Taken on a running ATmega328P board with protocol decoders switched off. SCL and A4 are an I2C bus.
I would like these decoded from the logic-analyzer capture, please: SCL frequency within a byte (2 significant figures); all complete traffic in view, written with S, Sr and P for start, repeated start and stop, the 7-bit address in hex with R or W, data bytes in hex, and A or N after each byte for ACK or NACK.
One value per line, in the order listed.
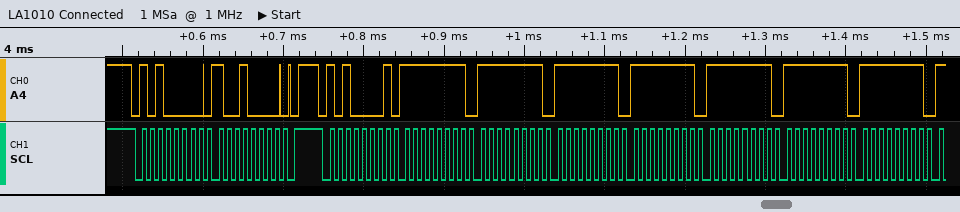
100 kHz
S 50W A 90 A P S 50R A FF A FF A FF A FF A FF A FF A FF A
